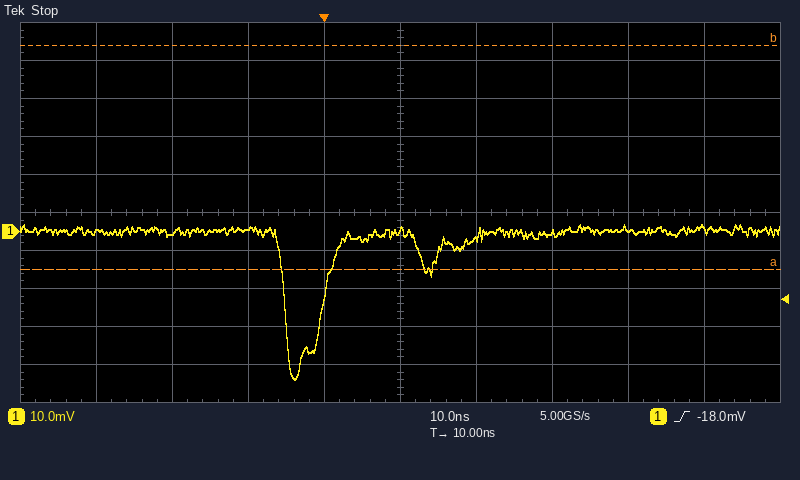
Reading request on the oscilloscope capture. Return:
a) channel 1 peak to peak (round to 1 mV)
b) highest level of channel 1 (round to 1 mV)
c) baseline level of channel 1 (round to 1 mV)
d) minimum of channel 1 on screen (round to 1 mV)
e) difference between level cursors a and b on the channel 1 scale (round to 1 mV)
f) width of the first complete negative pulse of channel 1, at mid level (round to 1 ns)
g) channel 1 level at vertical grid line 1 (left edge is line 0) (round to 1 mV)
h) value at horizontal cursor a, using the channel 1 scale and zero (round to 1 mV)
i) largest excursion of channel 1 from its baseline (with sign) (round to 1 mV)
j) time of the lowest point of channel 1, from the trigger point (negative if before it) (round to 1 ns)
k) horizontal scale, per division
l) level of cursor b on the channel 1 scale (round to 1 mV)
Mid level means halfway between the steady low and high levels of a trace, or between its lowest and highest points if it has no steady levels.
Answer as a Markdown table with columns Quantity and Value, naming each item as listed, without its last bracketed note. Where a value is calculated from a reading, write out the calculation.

| Quantity | Value |
|---|---|
| channel 1 peak to peak | 2 mV − (-39 mV) = 41 mV |
| highest level of channel 1 | 2 mV |
| baseline level of channel 1 | 0 mV |
| minimum of channel 1 on screen | -39 mV |
| difference between level cursors a and b on the channel 1 scale | 59 mV |
| width of the first complete negative pulse of channel 1, at mid level | 5 ns |
| channel 1 level at vertical grid line 1 (left edge is line 0) | 0 mV |
| value at horizontal cursor a, using the channel 1 scale and zero | -10 mV |
| largest excursion of channel 1 from its baseline (with sign) | -39 mV − (0 mV) = -39 mV |
| time of the lowest point of channel 1, from the trigger point (negative if before it) | -4 ns |
| horizontal scale, per division | 10 ns |
| level of cursor b on the channel 1 scale | 49 mV |
